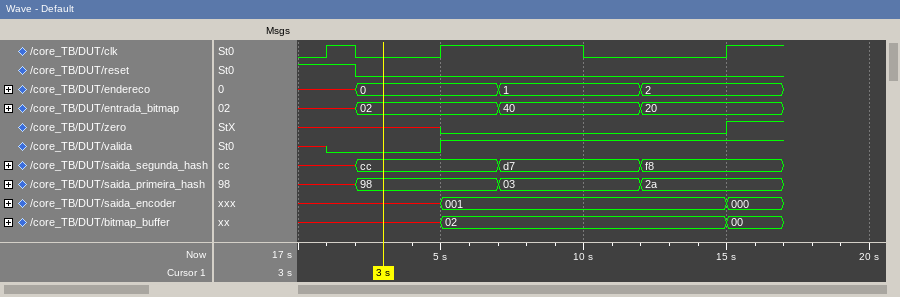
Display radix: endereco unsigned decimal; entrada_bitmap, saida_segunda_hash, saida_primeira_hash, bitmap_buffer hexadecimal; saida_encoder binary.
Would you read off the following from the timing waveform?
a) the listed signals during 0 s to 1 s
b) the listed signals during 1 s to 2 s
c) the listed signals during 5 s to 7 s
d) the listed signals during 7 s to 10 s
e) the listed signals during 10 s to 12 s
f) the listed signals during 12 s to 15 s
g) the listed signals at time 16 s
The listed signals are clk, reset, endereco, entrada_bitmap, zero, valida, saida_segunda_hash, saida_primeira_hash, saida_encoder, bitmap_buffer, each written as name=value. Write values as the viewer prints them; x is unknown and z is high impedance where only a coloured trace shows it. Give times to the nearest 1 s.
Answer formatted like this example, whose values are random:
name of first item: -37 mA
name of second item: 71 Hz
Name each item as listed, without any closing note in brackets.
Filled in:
the listed signals during 0 s to 1 s: clk=0, reset=1, endereco=x, entrada_bitmap=x, zero=x, valida=x, saida_segunda_hash=x, saida_primeira_hash=x, saida_encoder=x, bitmap_buffer=x
the listed signals during 1 s to 2 s: clk=1, reset=1, endereco=x, entrada_bitmap=x, zero=x, valida=0, saida_segunda_hash=x, saida_primeira_hash=x, saida_encoder=x, bitmap_buffer=x
the listed signals during 5 s to 7 s: clk=1, reset=0, endereco=0, entrada_bitmap=02, zero=0, valida=1, saida_segunda_hash=cc, saida_primeira_hash=98, saida_encoder=001, bitmap_buffer=02
the listed signals during 7 s to 10 s: clk=1, reset=0, endereco=1, entrada_bitmap=40, zero=0, valida=1, saida_segunda_hash=d7, saida_primeira_hash=03, saida_encoder=001, bitmap_buffer=02
the listed signals during 10 s to 12 s: clk=0, reset=0, endereco=1, entrada_bitmap=40, zero=0, valida=1, saida_segunda_hash=d7, saida_primeira_hash=03, saida_encoder=001, bitmap_buffer=02
the listed signals during 12 s to 15 s: clk=0, reset=0, endereco=2, entrada_bitmap=20, zero=0, valida=1, saida_segunda_hash=f8, saida_primeira_hash=2a, saida_encoder=001, bitmap_buffer=02
the listed signals at time 16 s: clk=1, reset=0, endereco=2, entrada_bitmap=20, zero=1, valida=1, saida_segunda_hash=f8, saida_primeira_hash=2a, saida_encoder=000, bitmap_buffer=00
